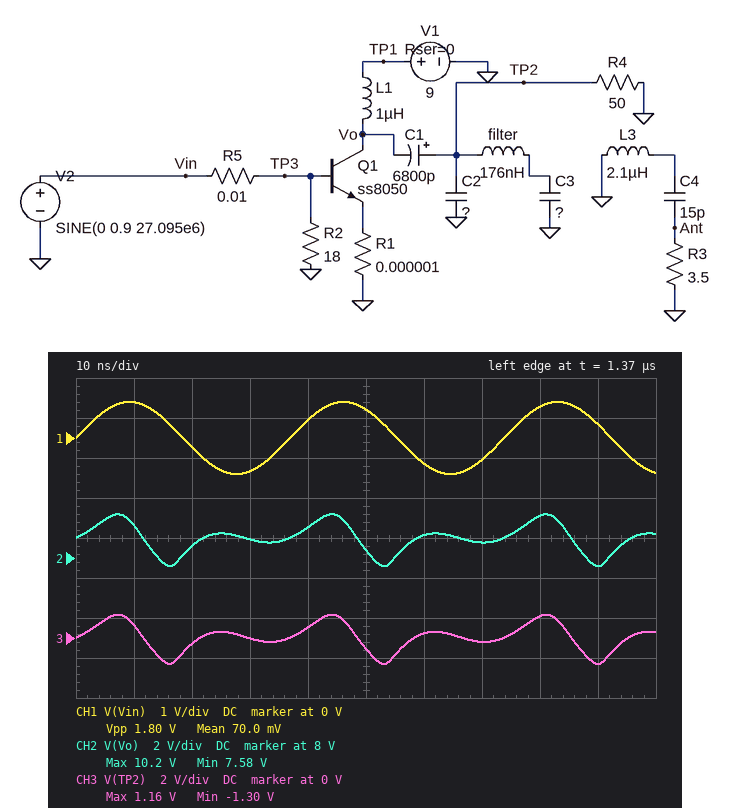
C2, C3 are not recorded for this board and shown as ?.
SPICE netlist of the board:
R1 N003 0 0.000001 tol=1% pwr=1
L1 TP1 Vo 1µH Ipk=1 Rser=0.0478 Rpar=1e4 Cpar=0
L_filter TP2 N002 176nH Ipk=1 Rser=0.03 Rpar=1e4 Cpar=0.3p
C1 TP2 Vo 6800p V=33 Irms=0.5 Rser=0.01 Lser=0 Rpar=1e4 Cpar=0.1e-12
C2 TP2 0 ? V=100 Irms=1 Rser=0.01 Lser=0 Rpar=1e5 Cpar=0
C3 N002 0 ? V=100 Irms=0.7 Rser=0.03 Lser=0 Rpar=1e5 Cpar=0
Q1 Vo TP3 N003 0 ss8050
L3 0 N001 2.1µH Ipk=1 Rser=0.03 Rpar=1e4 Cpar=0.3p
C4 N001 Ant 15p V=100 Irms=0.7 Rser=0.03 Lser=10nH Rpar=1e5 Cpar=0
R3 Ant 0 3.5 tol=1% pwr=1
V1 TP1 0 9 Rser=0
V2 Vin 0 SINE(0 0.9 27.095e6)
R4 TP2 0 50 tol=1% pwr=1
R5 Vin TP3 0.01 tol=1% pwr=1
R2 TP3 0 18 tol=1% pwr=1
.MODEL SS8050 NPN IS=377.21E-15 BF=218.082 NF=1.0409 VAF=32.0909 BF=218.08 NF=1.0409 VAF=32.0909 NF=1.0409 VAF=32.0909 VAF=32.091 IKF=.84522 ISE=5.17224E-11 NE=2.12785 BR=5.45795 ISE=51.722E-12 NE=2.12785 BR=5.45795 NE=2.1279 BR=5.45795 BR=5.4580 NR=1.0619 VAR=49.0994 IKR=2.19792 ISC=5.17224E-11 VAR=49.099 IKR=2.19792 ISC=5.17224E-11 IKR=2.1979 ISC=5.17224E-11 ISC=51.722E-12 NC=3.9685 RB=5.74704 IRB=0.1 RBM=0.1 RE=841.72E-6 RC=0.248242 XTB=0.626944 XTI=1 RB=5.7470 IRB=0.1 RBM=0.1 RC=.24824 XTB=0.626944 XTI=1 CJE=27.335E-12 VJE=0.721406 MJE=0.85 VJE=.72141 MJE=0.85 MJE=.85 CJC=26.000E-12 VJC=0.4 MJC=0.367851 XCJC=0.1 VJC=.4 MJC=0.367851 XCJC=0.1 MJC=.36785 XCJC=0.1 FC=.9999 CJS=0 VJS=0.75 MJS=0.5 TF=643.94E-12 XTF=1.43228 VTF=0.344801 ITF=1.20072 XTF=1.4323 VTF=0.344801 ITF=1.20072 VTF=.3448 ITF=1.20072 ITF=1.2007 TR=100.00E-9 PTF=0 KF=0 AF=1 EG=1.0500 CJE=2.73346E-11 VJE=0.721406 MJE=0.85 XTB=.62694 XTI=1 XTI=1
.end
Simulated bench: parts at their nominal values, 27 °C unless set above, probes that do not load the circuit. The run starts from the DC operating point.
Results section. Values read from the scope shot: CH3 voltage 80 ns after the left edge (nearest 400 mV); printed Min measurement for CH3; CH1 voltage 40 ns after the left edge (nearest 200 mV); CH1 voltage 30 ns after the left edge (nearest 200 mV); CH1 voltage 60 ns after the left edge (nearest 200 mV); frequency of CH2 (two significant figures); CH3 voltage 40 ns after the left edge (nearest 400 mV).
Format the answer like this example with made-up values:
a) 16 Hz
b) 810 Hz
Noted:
a) 1.2 V
b) -1.30 V
c) 400 mV
d) -800 mV
e) -600 mV
f) 27 MHz
g) 400 mV
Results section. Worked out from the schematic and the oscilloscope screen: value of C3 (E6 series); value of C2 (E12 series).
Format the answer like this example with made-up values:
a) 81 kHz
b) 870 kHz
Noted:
a) 150 pF
b) 270 pF
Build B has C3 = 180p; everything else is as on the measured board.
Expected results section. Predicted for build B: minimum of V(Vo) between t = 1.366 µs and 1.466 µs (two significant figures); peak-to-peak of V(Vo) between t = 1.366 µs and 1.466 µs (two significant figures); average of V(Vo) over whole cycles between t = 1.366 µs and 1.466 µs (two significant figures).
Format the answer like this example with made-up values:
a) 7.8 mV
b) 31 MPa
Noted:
a) 7.8 V
b) 2.2 V
c) 9.0 V
